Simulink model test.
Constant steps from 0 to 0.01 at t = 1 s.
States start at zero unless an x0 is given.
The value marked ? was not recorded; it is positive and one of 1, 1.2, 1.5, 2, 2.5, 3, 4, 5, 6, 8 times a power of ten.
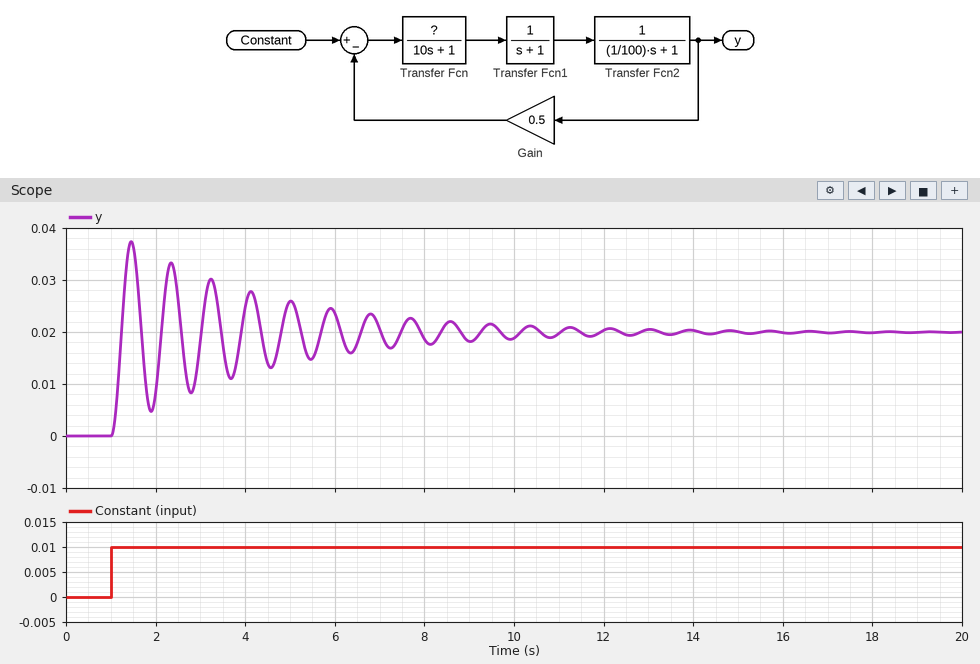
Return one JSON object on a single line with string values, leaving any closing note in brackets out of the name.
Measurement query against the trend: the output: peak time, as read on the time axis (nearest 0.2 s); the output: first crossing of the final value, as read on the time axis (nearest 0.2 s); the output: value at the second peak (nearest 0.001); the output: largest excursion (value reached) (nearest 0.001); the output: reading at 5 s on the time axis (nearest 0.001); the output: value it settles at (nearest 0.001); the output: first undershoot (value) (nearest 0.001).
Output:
{"the output: peak time, as read on the time axis": "1.4 s", "the output: first crossing of the final value, as read on the time axis": "1.2 s", "the output: value at the second peak": "0.033", "the output: largest excursion (value reached)": "0.037", "the output: reading at 5 s on the time axis": "0.026", "the output: value it settles at": "0.020", "the output: first undershoot (value)": "0.005"}
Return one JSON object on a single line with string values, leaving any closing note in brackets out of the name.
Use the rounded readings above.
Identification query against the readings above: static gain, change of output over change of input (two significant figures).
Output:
{"static gain, change of output over change of input": "2.0"}
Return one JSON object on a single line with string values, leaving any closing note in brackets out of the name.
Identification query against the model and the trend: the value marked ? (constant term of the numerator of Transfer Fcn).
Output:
{"the value marked ?": "1000"}
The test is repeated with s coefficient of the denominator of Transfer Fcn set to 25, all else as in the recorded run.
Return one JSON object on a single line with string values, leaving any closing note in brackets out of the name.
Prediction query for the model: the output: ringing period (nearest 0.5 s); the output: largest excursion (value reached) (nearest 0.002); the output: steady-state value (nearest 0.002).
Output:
{"the output: ringing period": "1.5 s", "the output: largest excursion (value reached)": "0.034", "the output: steady-state value": "0.020"}
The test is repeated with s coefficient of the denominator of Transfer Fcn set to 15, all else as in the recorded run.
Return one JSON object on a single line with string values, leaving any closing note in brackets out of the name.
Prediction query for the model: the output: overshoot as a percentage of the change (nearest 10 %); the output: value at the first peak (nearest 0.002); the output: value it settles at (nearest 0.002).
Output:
{"the output: overshoot as a percentage of the change": "80 %", "the output: value at the first peak": "0.036", "the output: value it settles at": "0.020"}
